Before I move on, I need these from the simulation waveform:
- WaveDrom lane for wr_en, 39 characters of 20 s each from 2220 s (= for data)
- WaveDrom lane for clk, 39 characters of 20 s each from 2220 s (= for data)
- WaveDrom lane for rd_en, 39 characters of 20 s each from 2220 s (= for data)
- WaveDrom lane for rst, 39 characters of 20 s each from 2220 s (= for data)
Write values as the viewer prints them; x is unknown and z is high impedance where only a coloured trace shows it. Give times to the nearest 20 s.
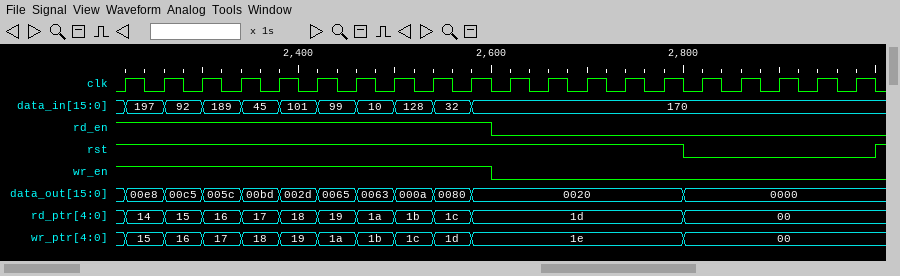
{name: 'wr_en', wave: '1..................0...................'}
{name: 'clk', wave: '101010101010101010101010101010101010101'}
{name: 'rd_en', wave: '1..................0...................'}
{name: 'rst', wave: '1............................0.........'}
